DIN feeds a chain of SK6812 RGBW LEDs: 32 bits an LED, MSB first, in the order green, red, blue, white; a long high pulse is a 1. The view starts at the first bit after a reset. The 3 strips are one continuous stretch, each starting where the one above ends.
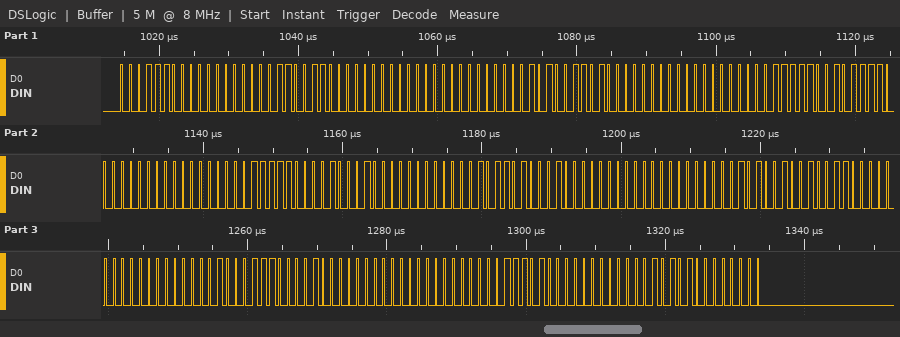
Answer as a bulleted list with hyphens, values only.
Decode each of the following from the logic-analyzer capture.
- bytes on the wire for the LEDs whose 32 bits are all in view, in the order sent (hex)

- 1C 00 33 00 00 01 4D 00 00 1F 2F 00 00 3E 11 00 0B 44 00 00 29 26 00 00 47 08 00 00 3A 00 15 00
